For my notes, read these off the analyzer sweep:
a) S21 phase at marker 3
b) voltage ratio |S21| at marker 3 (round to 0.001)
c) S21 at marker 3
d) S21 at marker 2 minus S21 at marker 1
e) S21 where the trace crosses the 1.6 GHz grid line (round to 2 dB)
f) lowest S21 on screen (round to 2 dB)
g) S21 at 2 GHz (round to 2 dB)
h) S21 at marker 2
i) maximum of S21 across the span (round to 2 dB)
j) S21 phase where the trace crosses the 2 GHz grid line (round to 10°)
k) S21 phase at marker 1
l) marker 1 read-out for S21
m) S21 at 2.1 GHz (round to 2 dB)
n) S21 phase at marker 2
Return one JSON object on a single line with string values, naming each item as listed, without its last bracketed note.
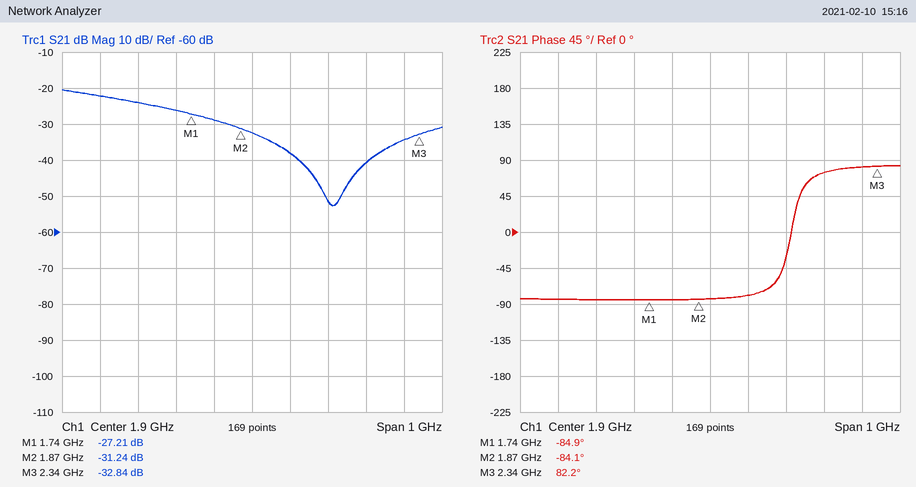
{"S21 phase at marker 3": "82.2°", "voltage ratio |S21| at marker 3": "0.023", "S21 at marker 3": "-32.84 dB", "S21 at marker 2 minus S21 at marker 1": "-4.03 dB", "S21 where the trace crosses the 1.6 GHz grid line": "-24 dB", "lowest S21 on screen": "-52 dB", "S21 at 2 GHz": "-38 dB", "S21 at marker 2": "-31.24 dB", "maximum of S21 across the span": "-20 dB", "S21 phase where the trace crosses the 2 GHz grid line": "-80°", "S21 phase at marker 1": "-84.9°", "marker 1 read-out for S21": "-27.21 dB", "S21 at 2.1 GHz": "-52 dB", "S21 phase at marker 2": "-84.1°"}
